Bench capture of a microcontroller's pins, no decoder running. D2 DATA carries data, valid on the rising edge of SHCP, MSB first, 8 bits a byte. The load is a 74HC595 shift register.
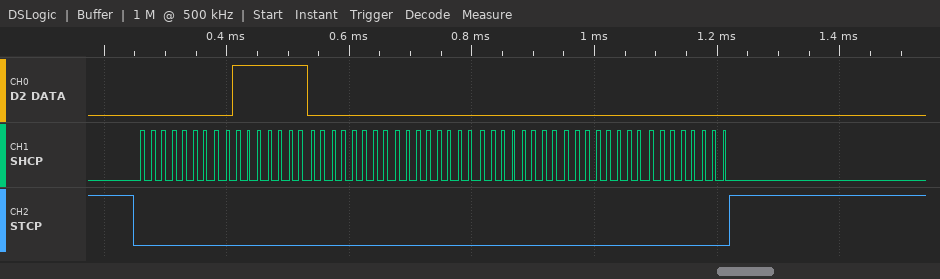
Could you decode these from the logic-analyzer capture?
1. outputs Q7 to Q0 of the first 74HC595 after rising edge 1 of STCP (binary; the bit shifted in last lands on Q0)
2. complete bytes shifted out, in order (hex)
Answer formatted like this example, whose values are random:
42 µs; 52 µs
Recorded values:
00000000; 00 7F 00 00 00 00 00
